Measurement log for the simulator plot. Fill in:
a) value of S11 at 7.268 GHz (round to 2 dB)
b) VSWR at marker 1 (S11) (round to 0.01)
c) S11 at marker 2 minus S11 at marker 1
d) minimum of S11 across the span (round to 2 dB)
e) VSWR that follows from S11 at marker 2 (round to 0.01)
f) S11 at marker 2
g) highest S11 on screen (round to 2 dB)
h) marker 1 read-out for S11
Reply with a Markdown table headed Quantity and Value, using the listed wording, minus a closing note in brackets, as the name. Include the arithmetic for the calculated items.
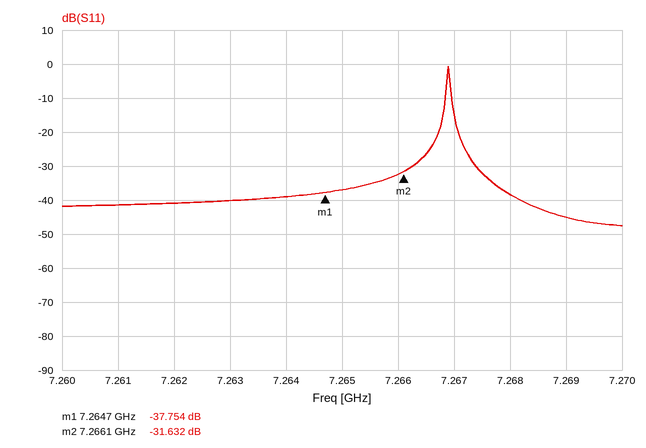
| Quantity | Value |
|---|---|
| value of S11 at 7.268 GHz | -38 dB |
| VSWR at marker 1 (S11) | (1 + 0.0130)/(1 − 0.0130) ≈ 1.03 |
| S11 at marker 2 minus S11 at marker 1 | -31.632 − (-37.754) = 6.122 dB |
| minimum of S11 across the span | -48 dB |
| VSWR that follows from S11 at marker 2 | (1 + 0.0262)/(1 − 0.0262) ≈ 1.05 |
| S11 at marker 2 | -31.632 dB |
| highest S11 on screen | 0 dB |
| marker 1 read-out for S11 | -37.754 dB |
